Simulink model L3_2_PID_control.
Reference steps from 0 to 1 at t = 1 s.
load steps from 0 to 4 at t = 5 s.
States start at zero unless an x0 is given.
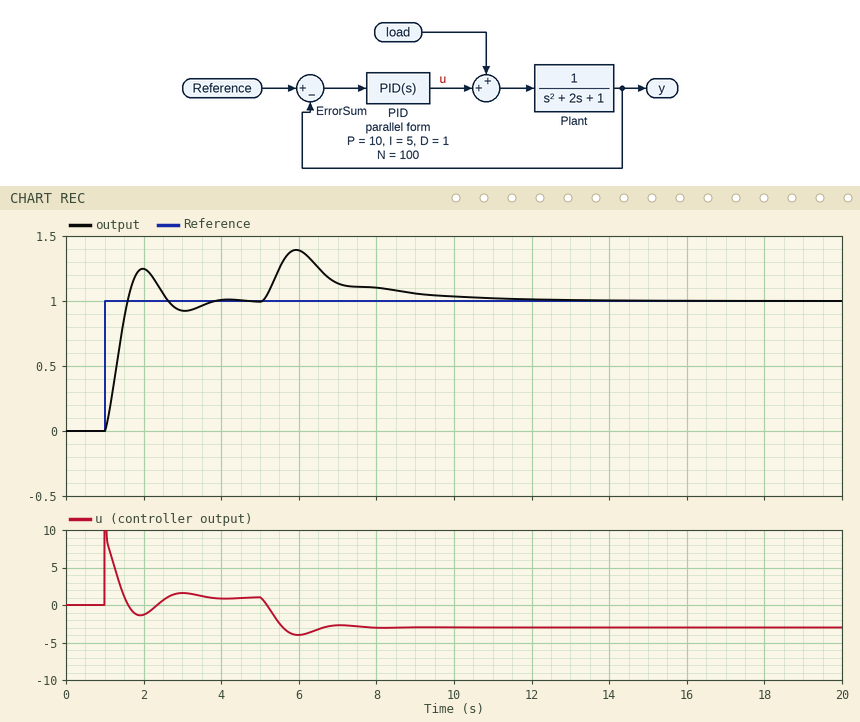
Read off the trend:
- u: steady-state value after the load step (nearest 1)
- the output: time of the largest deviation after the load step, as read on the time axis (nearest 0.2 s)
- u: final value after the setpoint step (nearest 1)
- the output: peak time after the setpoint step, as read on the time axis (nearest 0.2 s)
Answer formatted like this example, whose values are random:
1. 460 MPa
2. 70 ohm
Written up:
1. -3
2. 6.0 s
3. 1
4. 2.0 s
